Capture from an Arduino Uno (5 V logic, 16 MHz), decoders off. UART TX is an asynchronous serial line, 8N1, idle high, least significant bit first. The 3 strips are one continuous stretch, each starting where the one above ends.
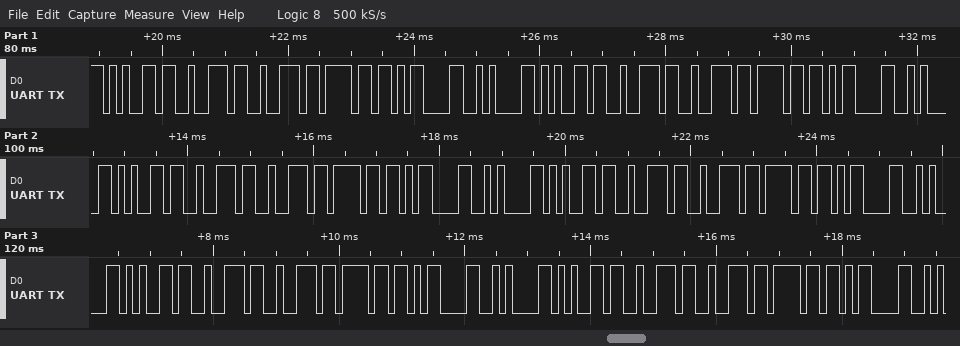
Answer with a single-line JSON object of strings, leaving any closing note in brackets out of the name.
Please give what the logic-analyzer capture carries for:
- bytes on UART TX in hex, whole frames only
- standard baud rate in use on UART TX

{"bytes on UART TX in hex, whole frames only": "0x65 0x72 0x72 0x6F 0x0D 0x0A 0x65 0x72 0x72 0x6F 0x0D 0x0A 0x65 0x72 0x72 0x6F 0x0D 0x0A 0x65 0x72 0x72 0x6F 0x0D 0x0A 0x65 0x72 0x72 0x6F 0x0D 0x0A 0x65 0x72 0x72 0x6F 0x0D", "standard baud rate in use on UART TX": "9600 baud"}
